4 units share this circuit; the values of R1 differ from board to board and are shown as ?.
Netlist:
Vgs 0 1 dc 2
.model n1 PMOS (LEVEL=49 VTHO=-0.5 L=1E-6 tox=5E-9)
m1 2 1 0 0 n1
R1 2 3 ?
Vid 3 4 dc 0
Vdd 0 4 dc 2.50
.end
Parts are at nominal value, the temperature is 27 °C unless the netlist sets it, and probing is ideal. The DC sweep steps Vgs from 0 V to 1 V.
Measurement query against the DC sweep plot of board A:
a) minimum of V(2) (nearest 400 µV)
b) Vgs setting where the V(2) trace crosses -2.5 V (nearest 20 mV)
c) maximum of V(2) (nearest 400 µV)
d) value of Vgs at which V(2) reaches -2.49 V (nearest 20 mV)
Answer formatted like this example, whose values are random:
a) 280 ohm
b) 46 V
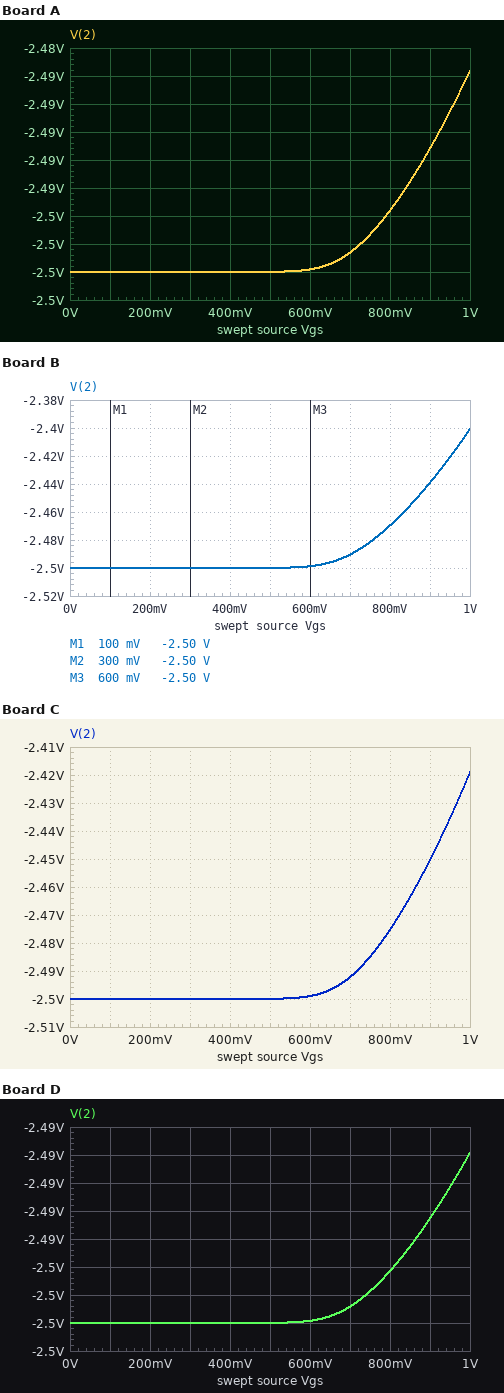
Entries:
a) -2.5000 V
b) 720 mV
c) -2.4856 V
d) 840 mV
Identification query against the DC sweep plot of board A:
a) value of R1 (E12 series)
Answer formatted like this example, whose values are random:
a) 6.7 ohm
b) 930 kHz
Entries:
a) 390 Ω
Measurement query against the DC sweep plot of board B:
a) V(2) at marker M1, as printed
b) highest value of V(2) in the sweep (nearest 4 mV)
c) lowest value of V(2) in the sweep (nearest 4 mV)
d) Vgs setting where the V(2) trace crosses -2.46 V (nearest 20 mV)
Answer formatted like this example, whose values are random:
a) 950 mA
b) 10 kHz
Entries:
a) -2.50 V
b) -2.400 V
c) -2.500 V
d) 840 mV
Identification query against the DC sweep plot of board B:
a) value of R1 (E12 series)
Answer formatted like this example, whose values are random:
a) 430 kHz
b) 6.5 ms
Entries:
a) 2.7 kΩ
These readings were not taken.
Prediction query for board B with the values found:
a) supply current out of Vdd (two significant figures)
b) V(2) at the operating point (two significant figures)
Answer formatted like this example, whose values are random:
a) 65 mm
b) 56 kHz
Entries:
a) 280 µA
b) -1.7 V
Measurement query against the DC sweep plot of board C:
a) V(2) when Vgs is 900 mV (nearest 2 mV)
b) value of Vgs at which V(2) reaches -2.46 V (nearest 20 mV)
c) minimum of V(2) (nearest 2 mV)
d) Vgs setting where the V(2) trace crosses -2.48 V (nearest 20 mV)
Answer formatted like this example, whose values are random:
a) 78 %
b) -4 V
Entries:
a) -2.450 V
b) 860 mV
c) -2.500 V
d) 780 mV
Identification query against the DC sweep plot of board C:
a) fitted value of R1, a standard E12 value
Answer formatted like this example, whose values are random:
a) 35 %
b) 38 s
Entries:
a) 2.2 kΩ
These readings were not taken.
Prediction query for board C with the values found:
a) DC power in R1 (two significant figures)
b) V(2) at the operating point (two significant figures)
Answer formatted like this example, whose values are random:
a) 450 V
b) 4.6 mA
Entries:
a) 180 µW
b) -1.9 V
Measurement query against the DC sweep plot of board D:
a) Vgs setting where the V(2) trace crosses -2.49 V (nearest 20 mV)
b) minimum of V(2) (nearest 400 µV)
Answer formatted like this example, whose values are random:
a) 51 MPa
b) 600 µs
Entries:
a) 960 mV
b) -2.5000 V
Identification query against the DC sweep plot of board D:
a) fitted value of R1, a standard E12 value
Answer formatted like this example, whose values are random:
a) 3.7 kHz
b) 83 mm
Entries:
a) 330 Ω
